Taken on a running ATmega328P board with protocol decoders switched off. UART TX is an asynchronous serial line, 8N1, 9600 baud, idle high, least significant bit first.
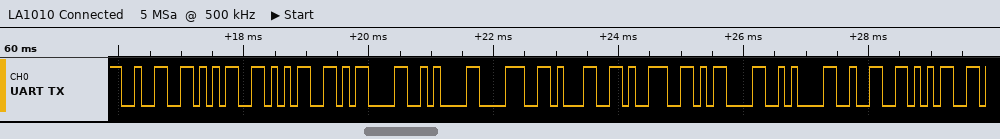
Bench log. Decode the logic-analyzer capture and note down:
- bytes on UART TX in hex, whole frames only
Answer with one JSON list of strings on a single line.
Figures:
["0x32 0x35 0x35 0x0D 0x0A 0x38 0x31 0x39 0x0D 0x0A 0x32 0x35"]
